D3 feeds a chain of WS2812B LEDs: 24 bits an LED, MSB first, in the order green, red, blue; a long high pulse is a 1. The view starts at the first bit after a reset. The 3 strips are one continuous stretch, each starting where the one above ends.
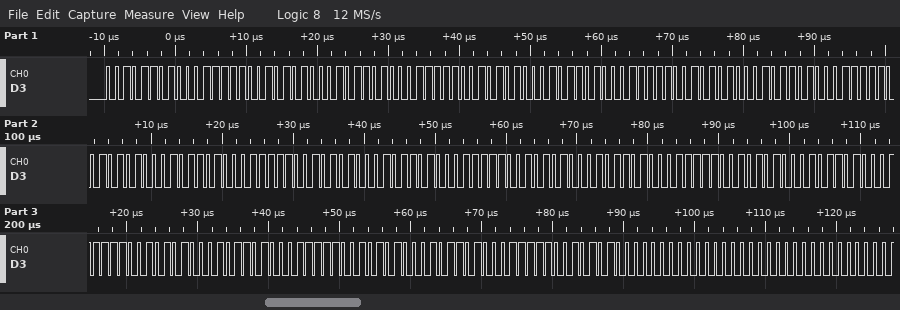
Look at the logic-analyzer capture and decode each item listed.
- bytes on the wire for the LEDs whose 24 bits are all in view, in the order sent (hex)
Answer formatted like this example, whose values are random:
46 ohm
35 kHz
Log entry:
2D 1F 2A 2D 1F 2A 2D 1F 2A 2D 1F 2A 2D 1F 2A 2D 1F 2A 2D 1F 2A 2D 1F 2A 2D 1F 2A 2D 1F 2A 00 00 00
